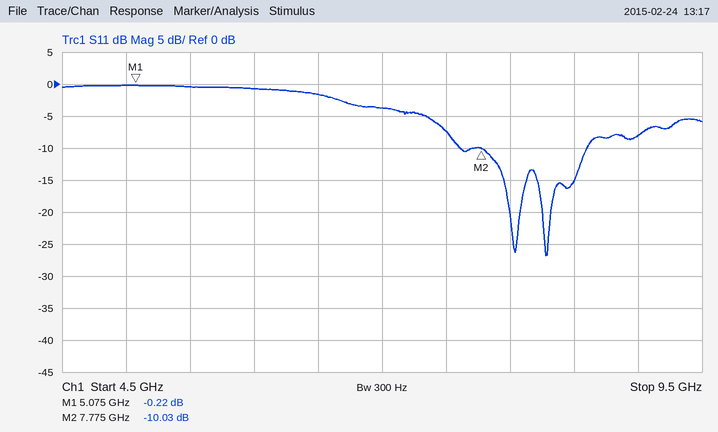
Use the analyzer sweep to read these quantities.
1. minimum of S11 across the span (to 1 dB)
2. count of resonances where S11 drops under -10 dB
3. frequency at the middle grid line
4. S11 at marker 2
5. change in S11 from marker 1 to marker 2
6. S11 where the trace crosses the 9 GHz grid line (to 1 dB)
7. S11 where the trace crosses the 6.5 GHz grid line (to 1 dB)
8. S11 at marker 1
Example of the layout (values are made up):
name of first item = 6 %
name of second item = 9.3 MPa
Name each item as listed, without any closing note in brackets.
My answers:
minimum of S11 across the span = -27 dB
count of resonances where S11 drops under -10 dB = 2
frequency at the middle grid line = 7 GHz
S11 at marker 2 = -10.03 dB
change in S11 from marker 1 to marker 2 = -9.81 dB
S11 where the trace crosses the 9 GHz grid line = -8 dB
S11 where the trace crosses the 6.5 GHz grid line = -2 dB
S11 at marker 1 = -0.22 dB
